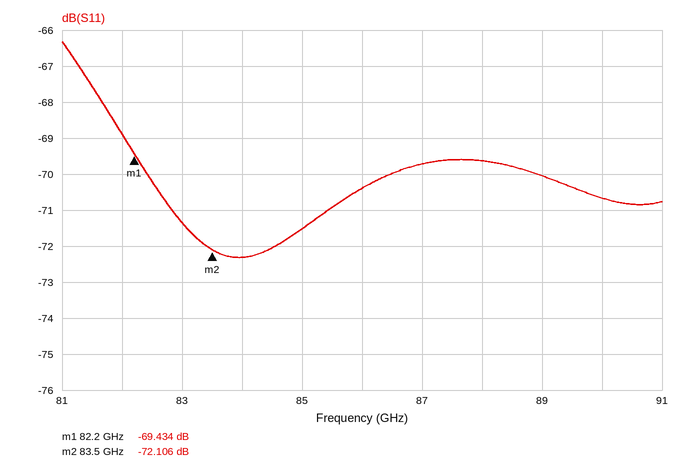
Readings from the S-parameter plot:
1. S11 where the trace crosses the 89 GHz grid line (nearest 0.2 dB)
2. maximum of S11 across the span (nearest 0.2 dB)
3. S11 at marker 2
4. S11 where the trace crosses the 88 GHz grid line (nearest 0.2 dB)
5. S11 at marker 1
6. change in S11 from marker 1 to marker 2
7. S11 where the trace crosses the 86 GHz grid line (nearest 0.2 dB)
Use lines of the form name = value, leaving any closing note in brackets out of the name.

S11 where the trace crosses the 89 GHz grid line = -70.0 dB
maximum of S11 across the span = -66.4 dB
S11 at marker 2 = -72.106 dB
S11 where the trace crosses the 88 GHz grid line = -69.6 dB
S11 at marker 1 = -69.434 dB
change in S11 from marker 1 to marker 2 = -2.672 dB
S11 where the trace crosses the 86 GHz grid line = -70.4 dB
